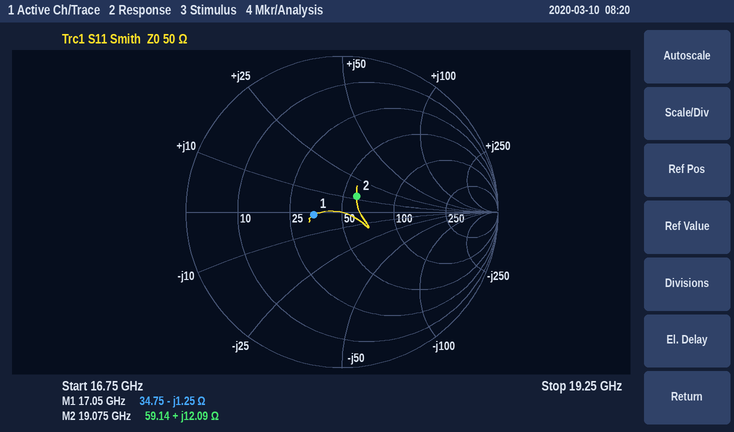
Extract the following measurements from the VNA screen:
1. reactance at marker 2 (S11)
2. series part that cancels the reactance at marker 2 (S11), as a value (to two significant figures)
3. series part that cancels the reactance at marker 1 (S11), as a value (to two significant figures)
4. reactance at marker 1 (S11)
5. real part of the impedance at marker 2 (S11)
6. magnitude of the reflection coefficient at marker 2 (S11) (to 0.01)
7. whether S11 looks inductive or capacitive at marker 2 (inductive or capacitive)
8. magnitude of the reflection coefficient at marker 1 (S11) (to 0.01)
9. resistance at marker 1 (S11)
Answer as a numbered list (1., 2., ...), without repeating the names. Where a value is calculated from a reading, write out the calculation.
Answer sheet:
1. +12.09 Ω
2. C = 1/(2π × 19.075 GHz × 12.09 Ω) ≈ 690 fF
3. L = 1.25 Ω/(2π × 17.05 GHz) ≈ 12 pH
4. -1.25 Ω
5. 59.14 Ω
6. 0.14
7. inductive
8. 0.18
9. 34.75 Ω
